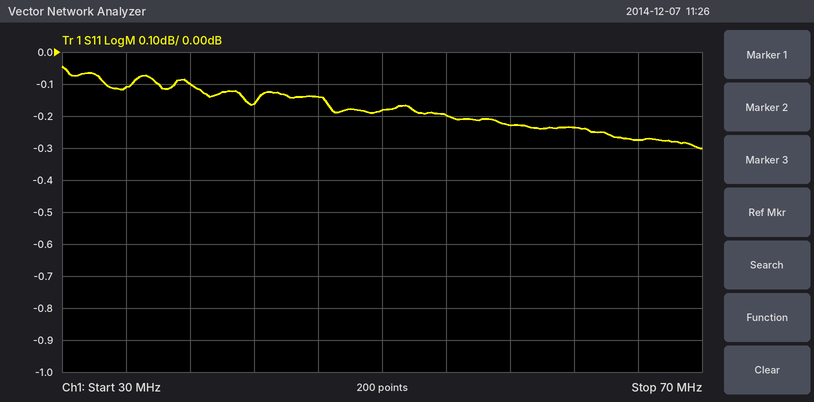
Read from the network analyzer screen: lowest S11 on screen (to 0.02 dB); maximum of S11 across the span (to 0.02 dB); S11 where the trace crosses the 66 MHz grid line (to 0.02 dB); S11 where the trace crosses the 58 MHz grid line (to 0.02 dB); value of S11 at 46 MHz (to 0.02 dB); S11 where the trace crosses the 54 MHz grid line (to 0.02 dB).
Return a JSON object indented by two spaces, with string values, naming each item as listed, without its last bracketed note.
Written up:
{
  "lowest S11 on screen": "-0.30 dB",
  "maximum of S11 across the span": "-0.04 dB",
  "S11 where the trace crosses the 66 MHz grid line": "-0.28 dB",
  "S11 where the trace crosses the 58 MHz grid line": "-0.22 dB",
  "value of S11 at 46 MHz": "-0.14 dB",
  "S11 where the trace crosses the 54 MHz grid line": "-0.20 dB"
}
